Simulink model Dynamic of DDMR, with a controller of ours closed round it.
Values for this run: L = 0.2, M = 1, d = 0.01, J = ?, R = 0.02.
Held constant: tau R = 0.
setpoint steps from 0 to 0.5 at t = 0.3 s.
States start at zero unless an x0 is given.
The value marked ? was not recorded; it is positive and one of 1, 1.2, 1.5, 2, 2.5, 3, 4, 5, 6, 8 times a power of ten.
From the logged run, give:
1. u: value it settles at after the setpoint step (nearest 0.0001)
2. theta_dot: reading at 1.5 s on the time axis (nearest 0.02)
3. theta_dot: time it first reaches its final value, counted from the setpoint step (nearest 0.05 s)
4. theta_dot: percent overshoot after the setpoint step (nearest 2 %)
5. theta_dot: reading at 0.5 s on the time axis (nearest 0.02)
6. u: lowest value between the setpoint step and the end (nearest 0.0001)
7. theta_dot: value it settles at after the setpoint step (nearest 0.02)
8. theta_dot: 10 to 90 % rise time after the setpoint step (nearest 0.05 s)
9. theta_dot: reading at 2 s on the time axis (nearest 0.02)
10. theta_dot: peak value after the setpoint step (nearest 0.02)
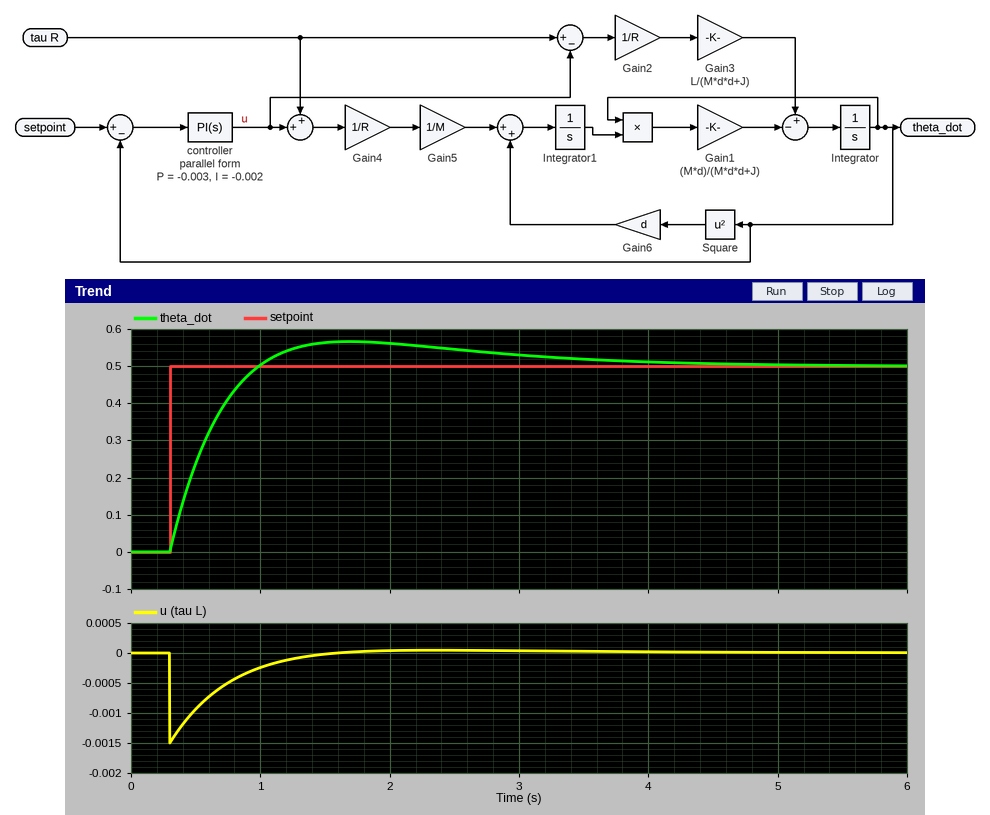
0.0000
0.56
0.70 s
14 %
0.24
-0.0015
0.50
0.50 s
0.56
0.56
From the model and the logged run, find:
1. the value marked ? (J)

0.01
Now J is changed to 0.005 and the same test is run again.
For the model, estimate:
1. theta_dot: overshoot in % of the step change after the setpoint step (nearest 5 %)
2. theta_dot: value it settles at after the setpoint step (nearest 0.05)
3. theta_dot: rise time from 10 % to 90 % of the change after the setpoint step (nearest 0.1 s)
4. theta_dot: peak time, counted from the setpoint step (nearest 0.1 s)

10 %
0.50
0.3 s
0.9 s
